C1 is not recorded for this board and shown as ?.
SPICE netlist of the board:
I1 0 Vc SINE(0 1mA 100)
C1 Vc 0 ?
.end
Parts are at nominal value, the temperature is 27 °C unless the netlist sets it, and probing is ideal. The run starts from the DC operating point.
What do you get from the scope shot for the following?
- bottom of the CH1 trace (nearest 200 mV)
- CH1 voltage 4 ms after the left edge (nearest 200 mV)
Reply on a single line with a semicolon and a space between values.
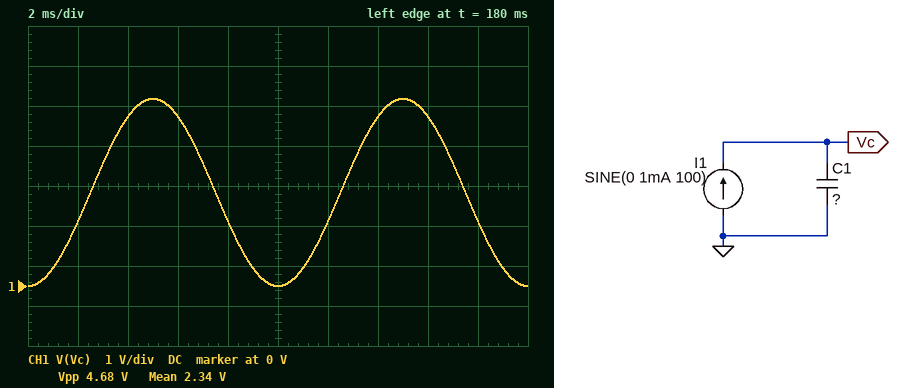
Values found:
0 V; 4.2 V
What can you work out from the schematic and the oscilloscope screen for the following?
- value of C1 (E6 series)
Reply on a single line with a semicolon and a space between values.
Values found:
680 nF
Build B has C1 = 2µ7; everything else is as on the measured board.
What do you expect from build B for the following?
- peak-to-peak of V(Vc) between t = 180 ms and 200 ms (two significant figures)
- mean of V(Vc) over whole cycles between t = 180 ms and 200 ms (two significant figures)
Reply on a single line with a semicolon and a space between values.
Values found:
1.2 V; 590 mV
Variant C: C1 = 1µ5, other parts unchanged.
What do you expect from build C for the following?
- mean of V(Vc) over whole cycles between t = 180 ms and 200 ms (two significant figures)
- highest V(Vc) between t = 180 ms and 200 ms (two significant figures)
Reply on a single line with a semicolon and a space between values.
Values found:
1.1 V; 2.1 V
